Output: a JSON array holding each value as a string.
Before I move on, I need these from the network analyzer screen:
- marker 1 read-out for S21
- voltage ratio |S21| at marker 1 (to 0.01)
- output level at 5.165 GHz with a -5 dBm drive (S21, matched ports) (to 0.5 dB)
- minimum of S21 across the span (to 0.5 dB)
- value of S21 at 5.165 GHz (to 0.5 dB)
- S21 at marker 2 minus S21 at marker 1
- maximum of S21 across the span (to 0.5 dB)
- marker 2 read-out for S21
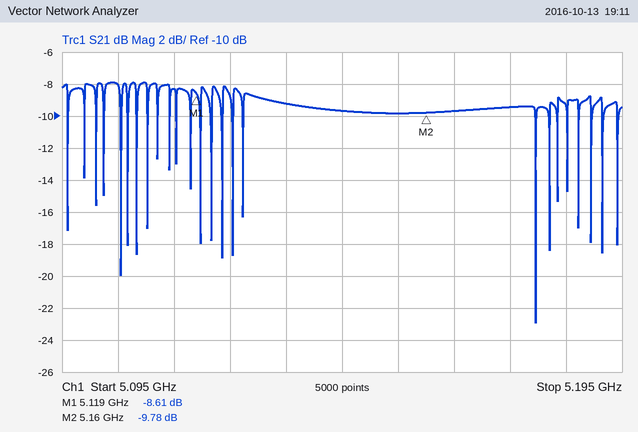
["-8.61 dB", "0.37", "-14.5 dBm", "-23.0 dB", "-9.5 dB", "-1.17 dB", "-8.0 dB", "-9.78 dB"]
